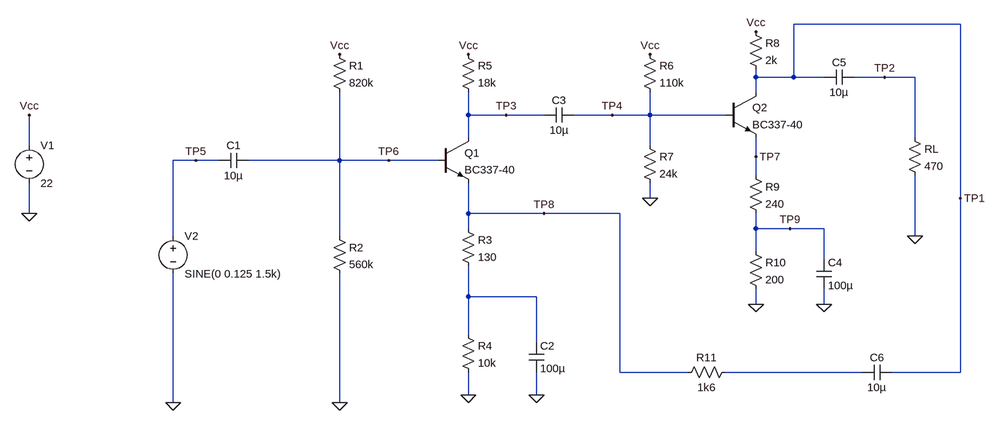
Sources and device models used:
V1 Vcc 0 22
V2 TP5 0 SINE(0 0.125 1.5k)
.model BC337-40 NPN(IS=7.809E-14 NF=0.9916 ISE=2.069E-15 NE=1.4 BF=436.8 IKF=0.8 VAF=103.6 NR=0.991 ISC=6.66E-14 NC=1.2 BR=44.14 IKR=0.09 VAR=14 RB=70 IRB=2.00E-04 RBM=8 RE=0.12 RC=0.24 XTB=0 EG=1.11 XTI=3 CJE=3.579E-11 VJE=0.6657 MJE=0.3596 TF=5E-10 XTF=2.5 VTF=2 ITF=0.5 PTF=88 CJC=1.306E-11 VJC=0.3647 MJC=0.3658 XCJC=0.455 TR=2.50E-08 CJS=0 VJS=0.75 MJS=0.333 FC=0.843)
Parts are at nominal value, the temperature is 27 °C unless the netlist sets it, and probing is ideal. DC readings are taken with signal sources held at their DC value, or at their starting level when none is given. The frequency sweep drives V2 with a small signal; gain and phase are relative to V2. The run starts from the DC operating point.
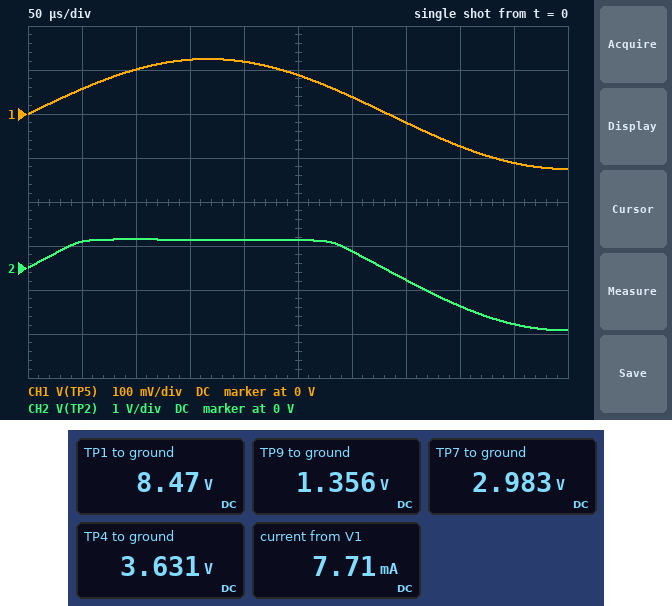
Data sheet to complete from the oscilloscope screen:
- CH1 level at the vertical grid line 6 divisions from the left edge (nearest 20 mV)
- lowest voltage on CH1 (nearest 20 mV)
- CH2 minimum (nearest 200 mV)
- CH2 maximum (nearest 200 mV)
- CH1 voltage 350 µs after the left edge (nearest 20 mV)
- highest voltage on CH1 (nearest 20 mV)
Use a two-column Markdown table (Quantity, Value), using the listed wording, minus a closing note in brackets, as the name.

| Quantity | Value |
|---|---|
| CH1 level at the vertical grid line 6 divisions from the left edge | 40 mV |
| lowest voltage on CH1 | -120 mV |
| CH2 minimum | -1.4 V |
| CH2 maximum | 600 mV |
| CH1 voltage 350 µs after the left edge | -20 mV |
| highest voltage on CH1 | 120 mV |
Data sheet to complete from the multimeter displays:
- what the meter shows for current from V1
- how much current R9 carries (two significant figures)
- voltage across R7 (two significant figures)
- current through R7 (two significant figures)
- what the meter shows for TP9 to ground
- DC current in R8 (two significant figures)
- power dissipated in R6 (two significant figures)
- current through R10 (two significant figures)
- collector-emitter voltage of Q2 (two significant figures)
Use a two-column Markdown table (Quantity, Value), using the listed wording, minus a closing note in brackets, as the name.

| Quantity | Value |
|---|---|
| what the meter shows for current from V1 | 7.71 mA |
| how much current R9 carries | 6.8 mA |
| voltage across R7 | 3.6 V |
| current through R7 | 150 µA |
| what the meter shows for TP9 to ground | 1.356 V |
| DC current in R8 | 6.8 mA |
| power dissipated in R6 | 3.1 mW |
| current through R10 | 6.8 mA |
| collector-emitter voltage of Q2 | 5.5 V |
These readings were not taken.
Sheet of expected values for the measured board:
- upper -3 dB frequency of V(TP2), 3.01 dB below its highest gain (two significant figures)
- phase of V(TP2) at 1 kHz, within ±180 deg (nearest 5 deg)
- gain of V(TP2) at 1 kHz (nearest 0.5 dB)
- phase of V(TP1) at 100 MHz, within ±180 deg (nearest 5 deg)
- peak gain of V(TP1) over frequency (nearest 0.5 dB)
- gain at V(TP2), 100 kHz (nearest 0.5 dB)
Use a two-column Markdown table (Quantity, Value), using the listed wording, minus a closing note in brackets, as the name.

| Quantity | Value |
|---|---|
| upper -3 dB frequency of V(TP2), 3.01 dB below its highest gain | 4.5 MHz |
| phase of V(TP2) at 1 kHz, within ±180 deg | 0 deg |
| gain of V(TP2) at 1 kHz | 21.0 dB |
| phase of V(TP1) at 100 MHz, within ±180 deg | 85 deg |
| peak gain of V(TP1) over frequency | 21.0 dB |
| gain at V(TP2), 100 kHz | 21.0 dB |
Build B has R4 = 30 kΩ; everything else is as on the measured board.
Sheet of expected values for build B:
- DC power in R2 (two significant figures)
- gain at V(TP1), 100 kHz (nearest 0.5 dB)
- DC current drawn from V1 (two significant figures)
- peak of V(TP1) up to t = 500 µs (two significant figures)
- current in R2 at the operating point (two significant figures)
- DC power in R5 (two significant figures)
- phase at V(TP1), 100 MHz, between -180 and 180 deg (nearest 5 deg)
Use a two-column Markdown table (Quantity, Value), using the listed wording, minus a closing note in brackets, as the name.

| Quantity | Value |
|---|---|
| DC power in R2 | 140 µW |
| gain at V(TP1), 100 kHz | 20.5 dB |
| DC current drawn from V1 | 7.2 mA |
| peak of V(TP1) up to t = 500 µs | 9.8 V |
| current in R2 at the operating point | 16 µA |
| DC power in R5 | 1.3 mW |
| phase at V(TP1), 100 MHz, between -180 and 180 deg | 95 deg |
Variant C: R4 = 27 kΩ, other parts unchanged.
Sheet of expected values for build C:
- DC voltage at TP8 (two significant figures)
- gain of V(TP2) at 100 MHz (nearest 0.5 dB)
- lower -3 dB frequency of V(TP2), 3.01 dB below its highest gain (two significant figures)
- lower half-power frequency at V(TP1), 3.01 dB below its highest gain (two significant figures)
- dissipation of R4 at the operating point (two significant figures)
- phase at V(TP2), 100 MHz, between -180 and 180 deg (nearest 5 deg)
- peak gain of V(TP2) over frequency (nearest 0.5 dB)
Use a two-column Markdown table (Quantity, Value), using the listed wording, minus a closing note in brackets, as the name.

| Quantity | Value |
|---|---|
| DC voltage at TP8 | 8.1 V |
| gain of V(TP2) at 100 MHz | -5.0 dB |
| lower -3 dB frequency of V(TP2), 3.01 dB below its highest gain | 32 Hz |
| lower half-power frequency at V(TP1), 3.01 dB below its highest gain | 350 mHz |
| dissipation of R4 at the operating point | 2.4 mW |
| phase at V(TP2), 100 MHz, between -180 and 180 deg | 95 deg |
| peak gain of V(TP2) over frequency | 20.5 dB |
